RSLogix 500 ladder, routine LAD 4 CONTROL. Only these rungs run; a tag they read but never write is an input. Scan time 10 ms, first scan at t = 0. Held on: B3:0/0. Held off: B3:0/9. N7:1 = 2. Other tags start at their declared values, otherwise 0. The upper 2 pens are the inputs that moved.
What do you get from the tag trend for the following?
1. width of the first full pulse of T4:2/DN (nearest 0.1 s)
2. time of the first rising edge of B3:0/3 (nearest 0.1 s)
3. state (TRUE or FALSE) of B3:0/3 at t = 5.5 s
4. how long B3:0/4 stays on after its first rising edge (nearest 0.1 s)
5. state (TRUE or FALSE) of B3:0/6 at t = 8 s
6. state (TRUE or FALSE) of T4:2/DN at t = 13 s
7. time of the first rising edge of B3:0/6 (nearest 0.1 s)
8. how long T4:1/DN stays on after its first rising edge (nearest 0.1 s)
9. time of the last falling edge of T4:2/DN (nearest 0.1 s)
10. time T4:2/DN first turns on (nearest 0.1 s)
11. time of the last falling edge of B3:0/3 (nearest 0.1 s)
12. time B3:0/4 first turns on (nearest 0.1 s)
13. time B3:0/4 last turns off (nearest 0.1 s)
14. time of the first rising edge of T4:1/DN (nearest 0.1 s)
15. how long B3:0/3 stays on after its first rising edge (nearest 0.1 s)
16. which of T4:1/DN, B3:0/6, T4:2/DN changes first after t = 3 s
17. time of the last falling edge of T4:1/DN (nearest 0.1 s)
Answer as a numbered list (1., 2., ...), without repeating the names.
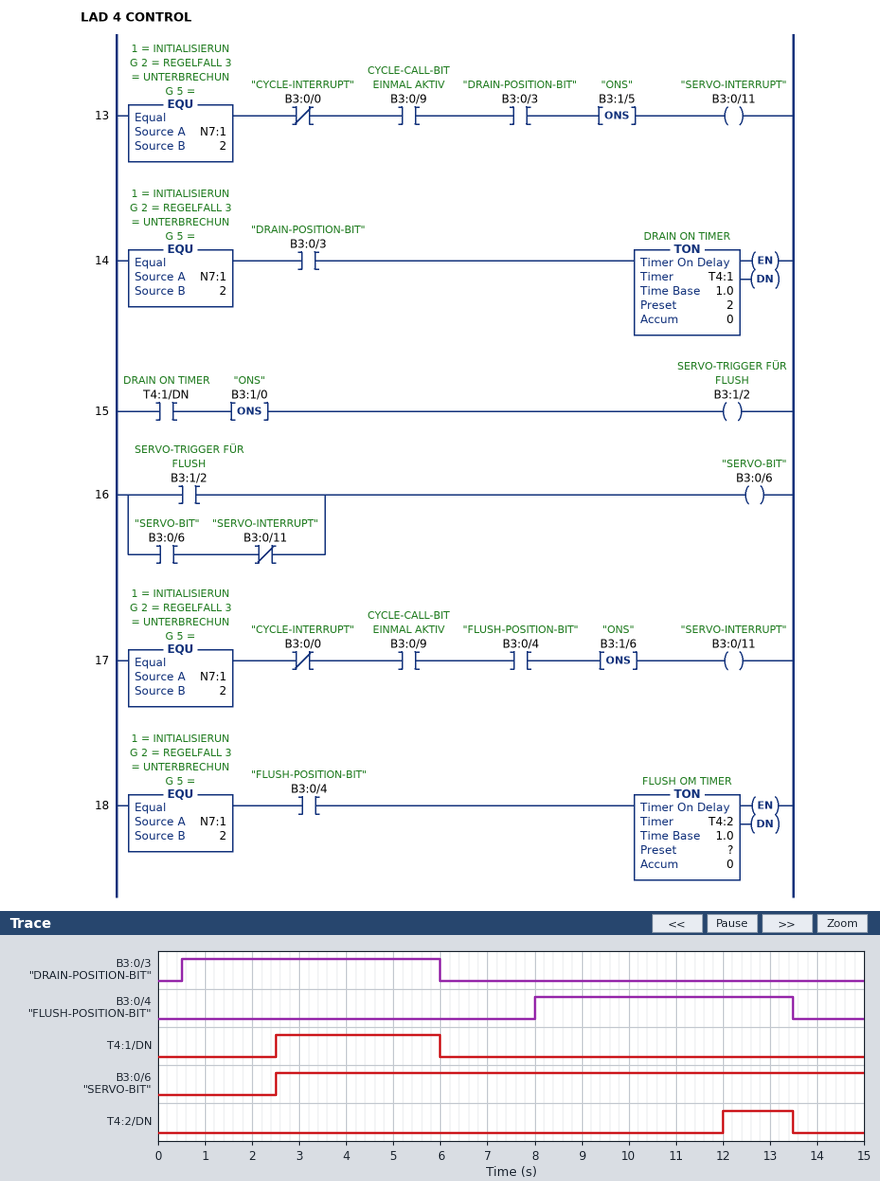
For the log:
1. 1.5 s
2. 0.5 s
3. TRUE
4. 5.5 s
5. TRUE
6. TRUE
7. 2.5 s
8. 3.5 s
9. 13.5 s
10. 12.0 s
11. 6.0 s
12. 8.0 s
13. 13.5 s
14. 2.5 s
15. 5.5 s
16. T4:1/DN
17. 6.0 s
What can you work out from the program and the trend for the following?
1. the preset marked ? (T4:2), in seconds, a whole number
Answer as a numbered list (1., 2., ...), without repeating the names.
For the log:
1. 4 s
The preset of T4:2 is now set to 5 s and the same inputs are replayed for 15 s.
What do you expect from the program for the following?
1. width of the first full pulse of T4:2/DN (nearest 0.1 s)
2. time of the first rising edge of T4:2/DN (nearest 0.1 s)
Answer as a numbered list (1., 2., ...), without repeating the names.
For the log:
1. 0.5 s
2. 13.0 s
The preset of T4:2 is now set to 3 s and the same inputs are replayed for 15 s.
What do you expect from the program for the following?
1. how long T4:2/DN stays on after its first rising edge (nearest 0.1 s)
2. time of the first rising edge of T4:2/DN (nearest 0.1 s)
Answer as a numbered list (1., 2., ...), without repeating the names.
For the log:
1. 2.5 s
2. 11.0 s
